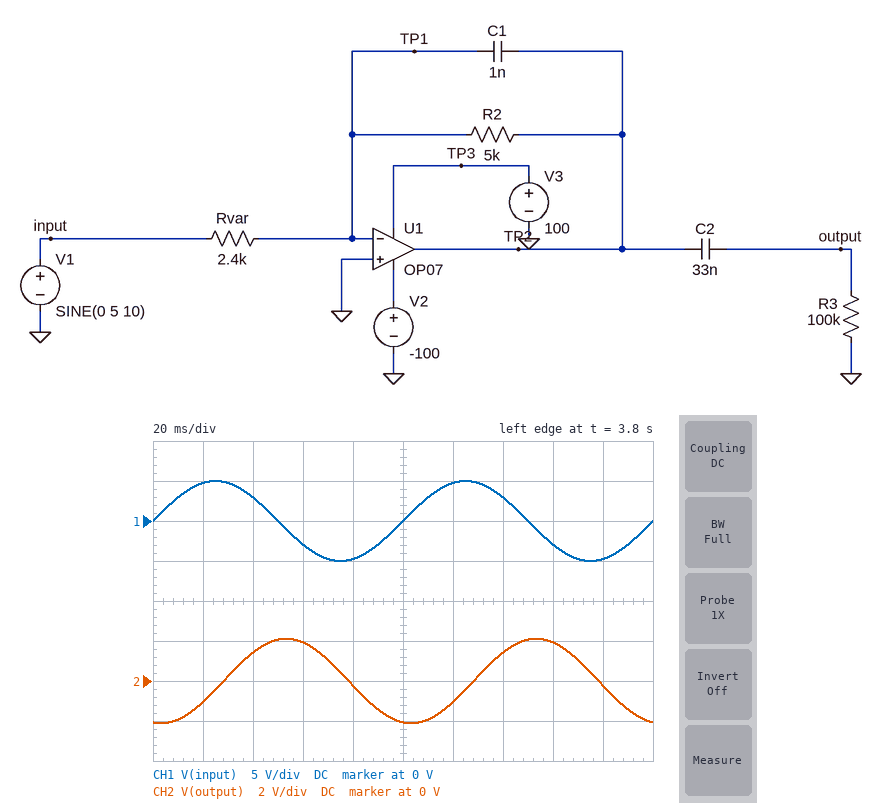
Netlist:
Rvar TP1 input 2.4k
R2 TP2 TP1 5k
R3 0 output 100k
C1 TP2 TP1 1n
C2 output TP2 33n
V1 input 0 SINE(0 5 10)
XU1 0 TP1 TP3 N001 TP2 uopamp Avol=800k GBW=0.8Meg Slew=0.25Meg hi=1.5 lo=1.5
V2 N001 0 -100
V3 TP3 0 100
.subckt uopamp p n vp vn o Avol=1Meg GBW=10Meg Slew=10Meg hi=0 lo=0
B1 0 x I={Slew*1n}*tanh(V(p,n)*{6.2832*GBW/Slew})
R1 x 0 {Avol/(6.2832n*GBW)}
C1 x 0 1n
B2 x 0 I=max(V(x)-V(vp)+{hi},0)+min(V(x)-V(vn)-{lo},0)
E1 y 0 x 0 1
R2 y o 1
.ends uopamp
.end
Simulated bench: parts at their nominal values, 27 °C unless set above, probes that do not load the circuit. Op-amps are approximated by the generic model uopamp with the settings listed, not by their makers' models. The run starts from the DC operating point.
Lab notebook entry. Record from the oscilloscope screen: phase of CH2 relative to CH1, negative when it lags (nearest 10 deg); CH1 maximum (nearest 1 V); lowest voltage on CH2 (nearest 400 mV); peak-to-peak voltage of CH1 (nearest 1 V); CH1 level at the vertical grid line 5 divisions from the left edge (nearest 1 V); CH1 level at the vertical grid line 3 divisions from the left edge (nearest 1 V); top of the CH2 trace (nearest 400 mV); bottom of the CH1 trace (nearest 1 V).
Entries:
-100 deg
5 V
-2.0 V
10 V
0 V
-3 V
2.0 V
-5 V
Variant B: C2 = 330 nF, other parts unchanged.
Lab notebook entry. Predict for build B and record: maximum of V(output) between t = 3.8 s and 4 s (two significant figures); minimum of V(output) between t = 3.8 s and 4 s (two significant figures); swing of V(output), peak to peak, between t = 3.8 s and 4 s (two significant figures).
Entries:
9.4 V
-9.4 V
19 V
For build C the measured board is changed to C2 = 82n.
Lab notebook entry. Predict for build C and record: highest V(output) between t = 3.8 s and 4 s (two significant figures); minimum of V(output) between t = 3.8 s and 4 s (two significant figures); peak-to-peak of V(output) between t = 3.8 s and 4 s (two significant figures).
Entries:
4.8 V
-4.8 V
9.5 V
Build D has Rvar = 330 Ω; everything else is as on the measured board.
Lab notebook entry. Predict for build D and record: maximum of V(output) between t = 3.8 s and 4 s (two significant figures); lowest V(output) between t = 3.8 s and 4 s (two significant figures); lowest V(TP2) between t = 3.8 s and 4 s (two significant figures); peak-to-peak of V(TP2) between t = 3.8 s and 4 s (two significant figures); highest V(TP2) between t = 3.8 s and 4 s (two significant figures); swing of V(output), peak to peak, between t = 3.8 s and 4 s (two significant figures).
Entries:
15 V
-15 V
-76 V
150 V
76 V
31 V
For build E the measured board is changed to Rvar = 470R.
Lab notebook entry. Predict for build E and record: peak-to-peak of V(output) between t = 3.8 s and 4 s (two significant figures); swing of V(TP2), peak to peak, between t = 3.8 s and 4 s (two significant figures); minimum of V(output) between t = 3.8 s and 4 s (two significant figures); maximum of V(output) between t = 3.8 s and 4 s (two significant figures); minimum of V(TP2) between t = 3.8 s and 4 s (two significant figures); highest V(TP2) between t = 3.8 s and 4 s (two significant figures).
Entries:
22 V
110 V
-11 V
11 V
-53 V
53 V
